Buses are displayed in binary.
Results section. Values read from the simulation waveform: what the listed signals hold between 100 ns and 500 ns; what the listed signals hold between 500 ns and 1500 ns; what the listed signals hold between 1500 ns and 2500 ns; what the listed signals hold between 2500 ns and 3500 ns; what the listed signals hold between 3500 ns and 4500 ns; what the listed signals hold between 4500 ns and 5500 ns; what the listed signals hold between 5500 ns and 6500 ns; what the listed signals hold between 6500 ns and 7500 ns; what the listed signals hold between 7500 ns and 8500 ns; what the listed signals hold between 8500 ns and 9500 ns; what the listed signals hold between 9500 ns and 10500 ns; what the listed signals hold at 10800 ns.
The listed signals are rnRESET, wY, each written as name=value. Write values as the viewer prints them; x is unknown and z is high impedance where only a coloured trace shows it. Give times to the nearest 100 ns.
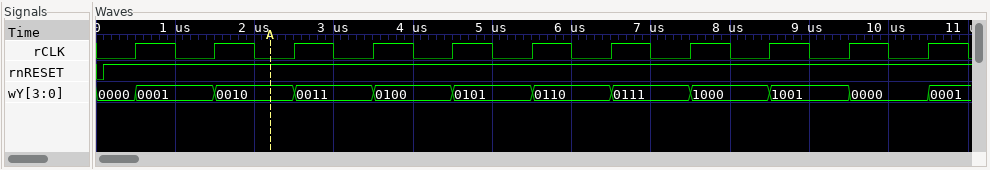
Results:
rnRESET=1, wY=0000
rnRESET=1, wY=0001
rnRESET=1, wY=0010
rnRESET=1, wY=0011
rnRESET=1, wY=0100
rnRESET=1, wY=0101
rnRESET=1, wY=0110
rnRESET=1, wY=0111
rnRESET=1, wY=1000
rnRESET=1, wY=1001
rnRESET=1, wY=0000
rnRESET=1, wY=0001
